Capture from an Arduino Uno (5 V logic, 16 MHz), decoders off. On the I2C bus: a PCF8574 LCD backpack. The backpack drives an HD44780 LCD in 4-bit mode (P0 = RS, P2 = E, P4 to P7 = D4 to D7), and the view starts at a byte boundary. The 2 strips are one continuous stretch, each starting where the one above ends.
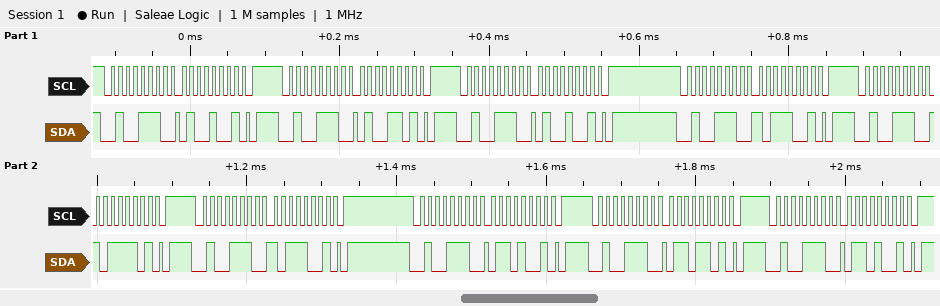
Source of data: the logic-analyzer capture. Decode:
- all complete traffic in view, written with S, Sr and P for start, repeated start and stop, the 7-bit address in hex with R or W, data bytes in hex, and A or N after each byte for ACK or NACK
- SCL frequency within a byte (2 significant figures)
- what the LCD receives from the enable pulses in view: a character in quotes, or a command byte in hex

S 27W A 49 A P S 27W A 4D A P S 27W A 49 A P S 27W A B9 A P S 27W A BD A P S 27W A B9 A P S 27W A 69 A P S 27W A 6D A P S 27W A 69 A P
100 kHz
'K'
